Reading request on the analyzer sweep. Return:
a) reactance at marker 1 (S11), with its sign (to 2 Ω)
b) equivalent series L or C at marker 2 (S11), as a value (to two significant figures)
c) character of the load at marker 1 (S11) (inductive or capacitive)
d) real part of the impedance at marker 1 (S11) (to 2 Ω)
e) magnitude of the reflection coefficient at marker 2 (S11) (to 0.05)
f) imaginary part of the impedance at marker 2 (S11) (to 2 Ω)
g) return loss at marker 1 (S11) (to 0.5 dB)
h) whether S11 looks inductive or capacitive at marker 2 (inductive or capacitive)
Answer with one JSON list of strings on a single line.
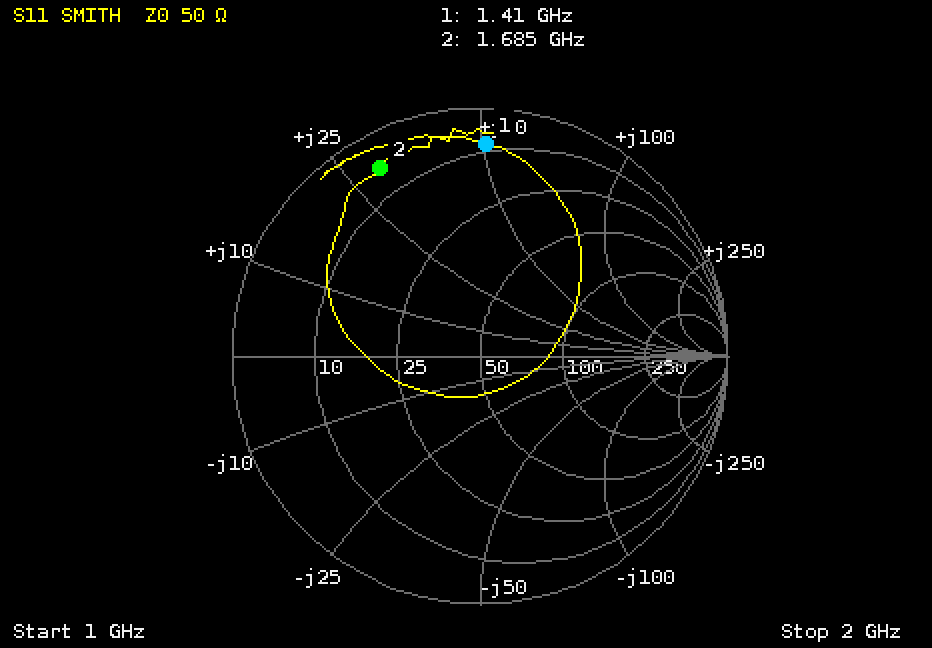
["+50 Ω", "2.8 nH", "inductive", "8 Ω", "0.85", "+30 Ω", "1.5 dB", "inductive"]
